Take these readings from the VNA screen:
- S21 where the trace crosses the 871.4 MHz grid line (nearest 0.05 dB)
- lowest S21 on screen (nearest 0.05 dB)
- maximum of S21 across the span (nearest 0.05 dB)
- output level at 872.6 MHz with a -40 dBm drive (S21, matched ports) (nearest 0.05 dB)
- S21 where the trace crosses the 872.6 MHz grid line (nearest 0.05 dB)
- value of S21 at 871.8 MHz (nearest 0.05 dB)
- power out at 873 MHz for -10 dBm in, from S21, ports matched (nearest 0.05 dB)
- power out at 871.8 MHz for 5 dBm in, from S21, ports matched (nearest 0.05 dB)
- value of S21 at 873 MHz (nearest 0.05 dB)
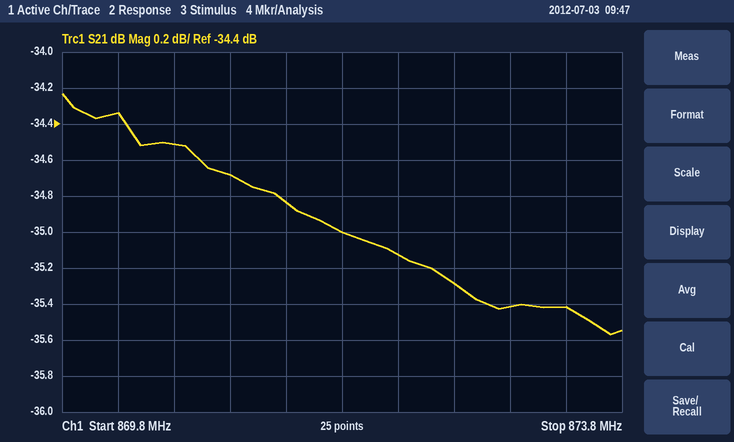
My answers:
-34.85 dB
-35.55 dB
-34.25 dB
-75.30 dBm
-35.30 dB
-35.00 dB
-45.40 dBm
-30.00 dBm
-35.40 dB
